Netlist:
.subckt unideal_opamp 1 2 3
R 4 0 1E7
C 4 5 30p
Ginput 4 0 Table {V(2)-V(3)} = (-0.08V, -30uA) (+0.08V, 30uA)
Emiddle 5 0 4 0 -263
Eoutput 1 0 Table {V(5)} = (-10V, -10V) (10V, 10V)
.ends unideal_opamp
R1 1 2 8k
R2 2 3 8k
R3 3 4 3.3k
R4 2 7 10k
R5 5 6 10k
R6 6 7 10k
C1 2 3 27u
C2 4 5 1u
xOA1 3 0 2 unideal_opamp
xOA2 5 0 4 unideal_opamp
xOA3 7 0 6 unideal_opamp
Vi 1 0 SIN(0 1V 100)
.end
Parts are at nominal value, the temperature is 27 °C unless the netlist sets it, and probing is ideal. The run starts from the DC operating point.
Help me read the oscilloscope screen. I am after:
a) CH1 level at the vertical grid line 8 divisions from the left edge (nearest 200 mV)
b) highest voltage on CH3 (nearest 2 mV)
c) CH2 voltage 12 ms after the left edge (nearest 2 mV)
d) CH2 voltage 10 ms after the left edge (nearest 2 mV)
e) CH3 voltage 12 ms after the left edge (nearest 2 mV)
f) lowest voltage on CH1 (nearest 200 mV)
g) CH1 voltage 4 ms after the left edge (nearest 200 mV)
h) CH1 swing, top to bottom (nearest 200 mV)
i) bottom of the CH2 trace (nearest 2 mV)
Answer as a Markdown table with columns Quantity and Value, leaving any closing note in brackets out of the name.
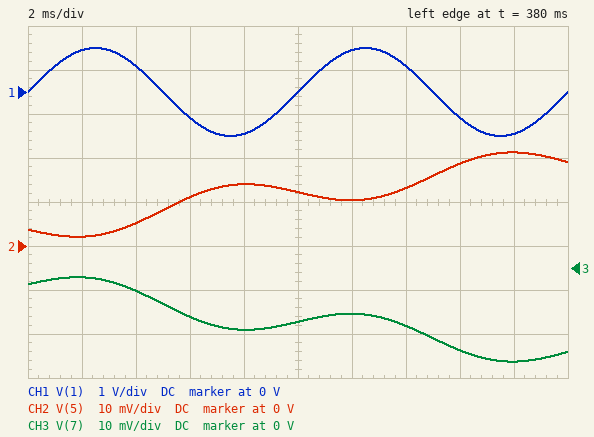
| Quantity | Value |
|---|---|
| CH1 level at the vertical grid line 8 divisions from the left edge | -600 mV |
| highest voltage on CH3 | -2 mV |
| CH2 voltage 12 ms after the left edge | 10 mV |
| CH2 voltage 10 ms after the left edge | 12 mV |
| CH3 voltage 12 ms after the left edge | -10 mV |
| lowest voltage on CH1 | -1.0 V |
| CH1 voltage 4 ms after the left edge | 600 mV |
| CH1 swing, top to bottom | 2.0 V |
| bottom of the CH2 trace | 2 mV |
